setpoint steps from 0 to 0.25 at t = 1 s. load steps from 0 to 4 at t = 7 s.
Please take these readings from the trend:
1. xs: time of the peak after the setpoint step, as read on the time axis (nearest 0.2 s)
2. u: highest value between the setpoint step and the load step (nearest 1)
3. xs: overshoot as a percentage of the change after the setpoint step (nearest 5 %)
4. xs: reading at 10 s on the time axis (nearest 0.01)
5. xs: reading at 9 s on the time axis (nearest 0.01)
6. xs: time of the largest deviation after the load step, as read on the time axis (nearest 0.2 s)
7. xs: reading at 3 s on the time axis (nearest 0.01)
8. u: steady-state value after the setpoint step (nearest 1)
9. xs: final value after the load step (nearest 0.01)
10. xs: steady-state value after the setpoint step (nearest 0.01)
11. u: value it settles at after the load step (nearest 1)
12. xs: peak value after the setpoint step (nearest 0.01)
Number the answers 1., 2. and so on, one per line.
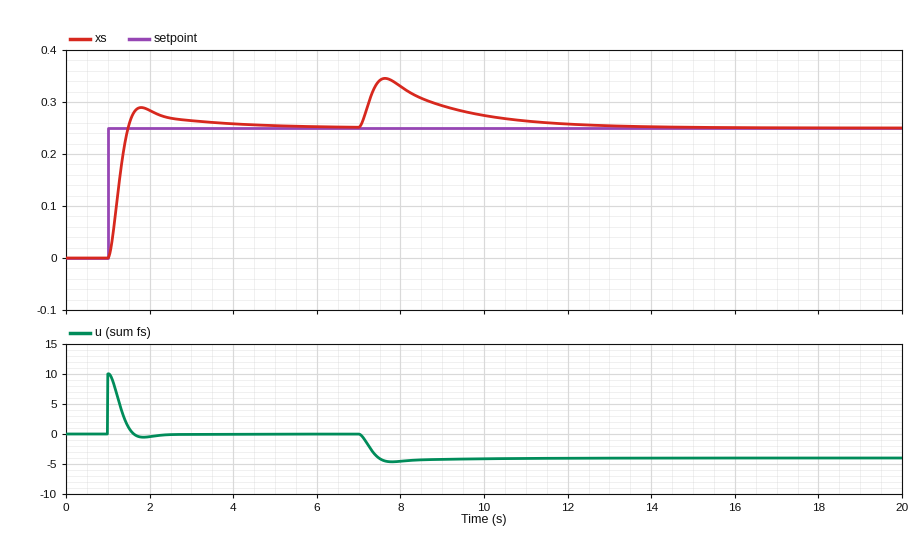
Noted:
1. 1.8 s
2. 10
3. 15 %
4. 0.27
5. 0.29
6. 7.6 s
7. 0.26
8. 0
9. 0.25
10. 0.25
11. -4
12. 0.29
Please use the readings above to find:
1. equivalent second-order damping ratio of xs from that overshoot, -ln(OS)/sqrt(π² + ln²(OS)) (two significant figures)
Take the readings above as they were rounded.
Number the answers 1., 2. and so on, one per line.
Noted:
1. 0.52
